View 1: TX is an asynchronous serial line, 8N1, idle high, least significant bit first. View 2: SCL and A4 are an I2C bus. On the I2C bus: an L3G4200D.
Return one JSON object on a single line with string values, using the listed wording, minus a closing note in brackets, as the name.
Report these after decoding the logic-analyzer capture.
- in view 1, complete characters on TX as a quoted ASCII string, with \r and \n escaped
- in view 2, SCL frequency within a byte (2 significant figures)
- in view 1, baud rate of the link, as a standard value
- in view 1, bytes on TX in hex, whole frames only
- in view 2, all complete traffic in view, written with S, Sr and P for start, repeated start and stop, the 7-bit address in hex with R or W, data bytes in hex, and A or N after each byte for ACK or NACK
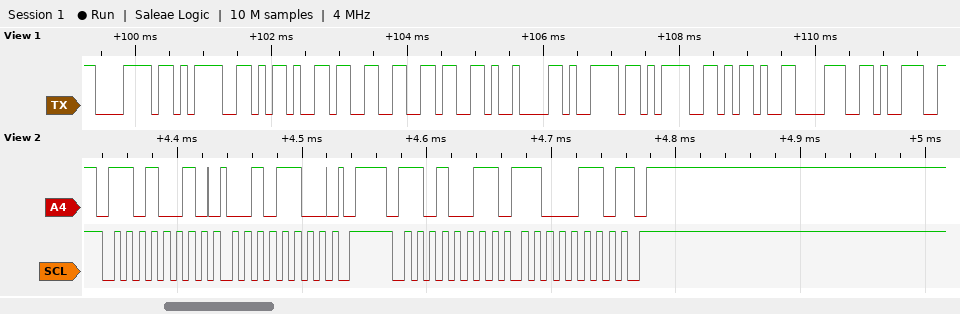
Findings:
{"in view 1, complete characters on TX as a quoted ASCII string, with \\r and \\n escaped": "\"x=-36\\ty=-89\"", "in view 2, SCL frequency within a byte": "100 kHz", "in view 1, baud rate of the link, as a standard value": "9600 baud", "in view 1, bytes on TX in hex, whole frames only": "78 3D 2D 33 36 09 79 3D 2D 38 39", "in view 2, all complete traffic in view, written with S, Sr and P for start, repeated start and stop, the 7-bit address in hex with R or W, data bytes in hex, and A or N after each byte for ACK or NACK": "S 69W A 2C A P S 69R A C6 N P"}
